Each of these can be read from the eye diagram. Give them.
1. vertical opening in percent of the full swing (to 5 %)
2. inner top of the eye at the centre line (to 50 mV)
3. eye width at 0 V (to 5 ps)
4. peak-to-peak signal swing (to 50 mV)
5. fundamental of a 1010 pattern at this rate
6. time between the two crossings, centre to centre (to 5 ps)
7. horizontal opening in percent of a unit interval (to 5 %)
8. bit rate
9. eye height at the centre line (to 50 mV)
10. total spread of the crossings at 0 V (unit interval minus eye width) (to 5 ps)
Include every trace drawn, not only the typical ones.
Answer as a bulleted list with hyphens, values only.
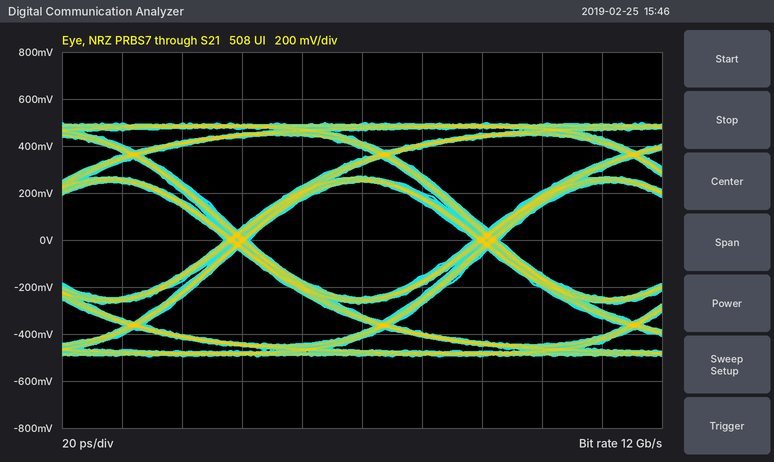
- 50 %
- 250 mV
- 75 ps
- 1.00 V
- 6 GHz
- 85 ps
- 90 %
- 12 Gb/s
- 500 mV
- 10 ps
